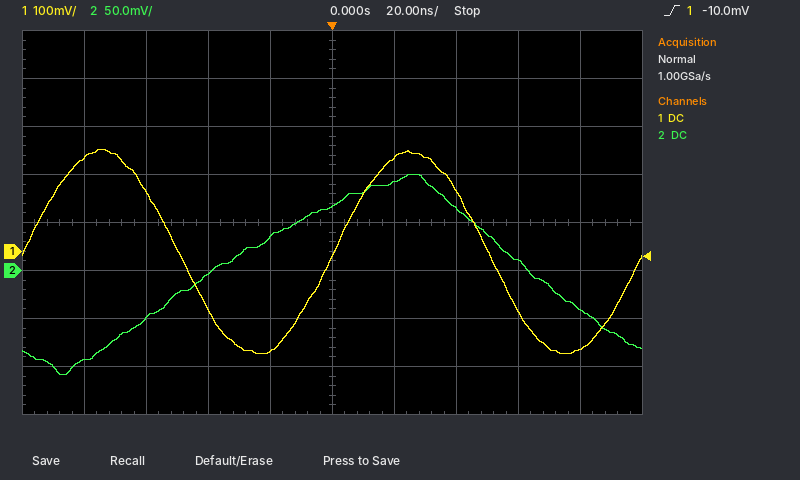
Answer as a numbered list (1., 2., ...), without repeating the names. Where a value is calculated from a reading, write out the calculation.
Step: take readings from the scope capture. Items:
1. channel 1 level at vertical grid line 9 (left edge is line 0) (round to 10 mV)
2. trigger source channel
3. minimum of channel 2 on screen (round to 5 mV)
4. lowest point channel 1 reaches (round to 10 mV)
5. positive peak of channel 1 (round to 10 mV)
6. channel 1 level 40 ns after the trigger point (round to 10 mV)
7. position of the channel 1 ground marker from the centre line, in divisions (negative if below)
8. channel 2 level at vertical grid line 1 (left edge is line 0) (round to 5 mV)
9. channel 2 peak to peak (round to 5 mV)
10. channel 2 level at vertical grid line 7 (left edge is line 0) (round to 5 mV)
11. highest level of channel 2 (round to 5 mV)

1. -200 mV
2. channel 1
3. -110 mV
4. -210 mV
5. 210 mV
6. 130 mV
7. -0.6 div
8. -95 mV
9. 100 mV − (-110 mV) = 210 mV
10. 65 mV
11. 100 mV
